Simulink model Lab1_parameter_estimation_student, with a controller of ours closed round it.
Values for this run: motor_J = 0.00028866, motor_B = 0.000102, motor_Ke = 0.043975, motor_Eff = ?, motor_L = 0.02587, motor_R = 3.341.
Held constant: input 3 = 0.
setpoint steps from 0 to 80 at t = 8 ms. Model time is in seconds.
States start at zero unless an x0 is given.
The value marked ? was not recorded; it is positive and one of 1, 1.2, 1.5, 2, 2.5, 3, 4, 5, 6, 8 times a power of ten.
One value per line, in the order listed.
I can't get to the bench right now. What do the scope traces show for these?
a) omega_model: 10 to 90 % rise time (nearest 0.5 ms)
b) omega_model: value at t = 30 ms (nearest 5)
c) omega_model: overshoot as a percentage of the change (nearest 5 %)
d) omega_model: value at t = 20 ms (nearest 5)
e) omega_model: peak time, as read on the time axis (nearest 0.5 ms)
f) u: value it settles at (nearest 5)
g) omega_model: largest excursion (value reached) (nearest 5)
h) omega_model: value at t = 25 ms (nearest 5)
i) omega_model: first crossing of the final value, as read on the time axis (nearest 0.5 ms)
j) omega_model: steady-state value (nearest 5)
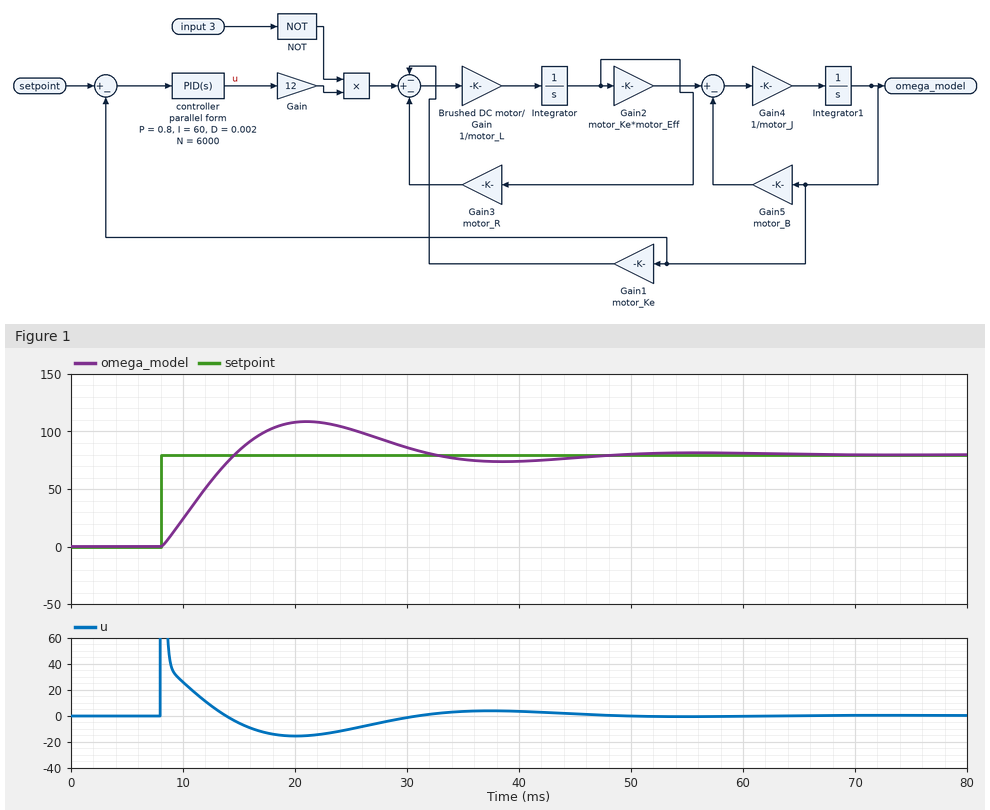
5.0 ms
85
35 %
110
21.0 ms
0
110
100
14.5 ms
80
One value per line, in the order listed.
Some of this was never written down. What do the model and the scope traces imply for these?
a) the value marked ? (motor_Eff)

1
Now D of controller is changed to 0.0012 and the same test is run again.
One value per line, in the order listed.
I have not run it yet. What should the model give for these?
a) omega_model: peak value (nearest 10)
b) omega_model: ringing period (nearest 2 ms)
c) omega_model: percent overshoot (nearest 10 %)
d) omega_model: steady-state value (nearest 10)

120
30 ms
50 %
80
